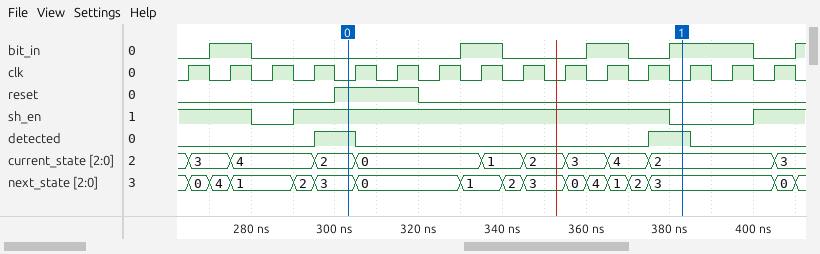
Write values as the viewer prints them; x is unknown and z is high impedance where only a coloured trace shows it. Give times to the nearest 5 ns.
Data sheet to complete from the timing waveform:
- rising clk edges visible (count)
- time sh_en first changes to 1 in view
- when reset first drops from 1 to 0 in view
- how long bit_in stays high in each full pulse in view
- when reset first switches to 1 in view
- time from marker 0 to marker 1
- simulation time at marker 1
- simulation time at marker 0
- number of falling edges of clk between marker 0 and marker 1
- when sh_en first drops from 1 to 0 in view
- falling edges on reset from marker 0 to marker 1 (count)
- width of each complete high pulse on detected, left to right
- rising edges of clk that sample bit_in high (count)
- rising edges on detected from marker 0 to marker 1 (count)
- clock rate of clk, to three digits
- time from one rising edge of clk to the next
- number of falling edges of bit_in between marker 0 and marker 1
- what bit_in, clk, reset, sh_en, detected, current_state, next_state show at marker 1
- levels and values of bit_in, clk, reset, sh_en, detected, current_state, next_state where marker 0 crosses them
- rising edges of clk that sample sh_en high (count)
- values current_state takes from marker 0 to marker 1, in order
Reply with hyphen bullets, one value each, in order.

- 15
- 290 ns
- 320 ns
- 10 ns, 10 ns, 10 ns, 20 ns
- 300 ns
- 80 ns
- 385 ns
- 305 ns
- 8
- 280 ns
- 1
- 10 ns, 10 ns
- 5
- 1
- 100 MHz
- 10 ns
- 2
- bit_in=1, clk=0, reset=0, sh_en=0, detected=1, current_state=2, next_state=3
- bit_in=0, clk=0, reset=1, sh_en=1, detected=1, current_state=2, next_state=3
- 12
- 2, 0, 1, 2, 3, 4, 2
